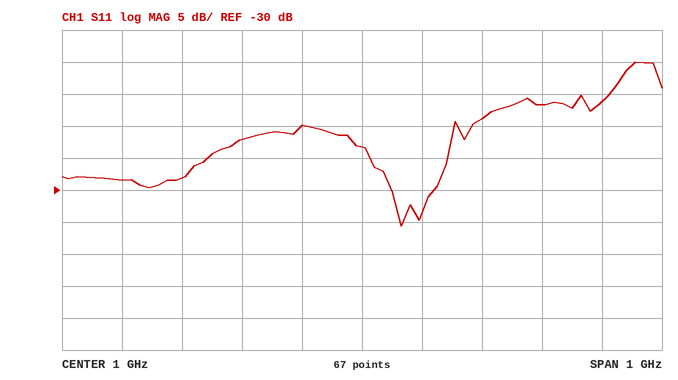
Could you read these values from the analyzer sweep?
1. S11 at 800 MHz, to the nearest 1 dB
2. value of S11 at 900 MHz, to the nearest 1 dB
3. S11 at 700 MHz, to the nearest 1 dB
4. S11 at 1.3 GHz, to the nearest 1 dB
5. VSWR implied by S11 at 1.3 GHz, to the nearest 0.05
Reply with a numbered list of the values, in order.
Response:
1. -22 dB
2. -20 dB
3. -28 dB
4. -17 dB
5. 1.35
